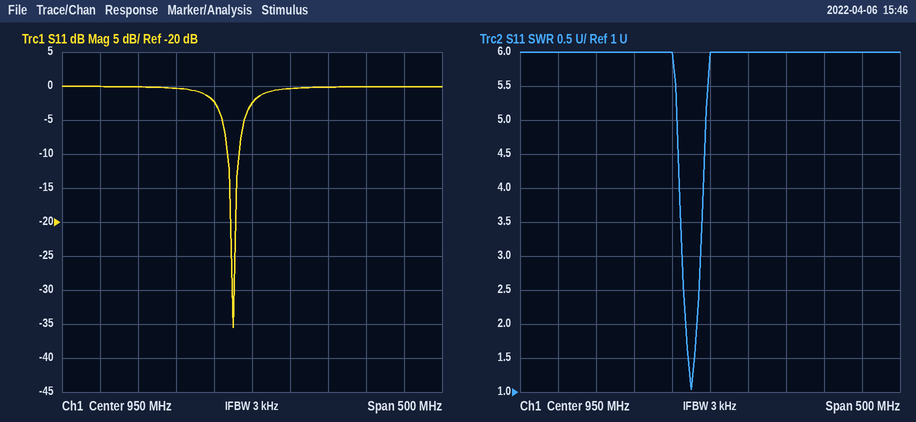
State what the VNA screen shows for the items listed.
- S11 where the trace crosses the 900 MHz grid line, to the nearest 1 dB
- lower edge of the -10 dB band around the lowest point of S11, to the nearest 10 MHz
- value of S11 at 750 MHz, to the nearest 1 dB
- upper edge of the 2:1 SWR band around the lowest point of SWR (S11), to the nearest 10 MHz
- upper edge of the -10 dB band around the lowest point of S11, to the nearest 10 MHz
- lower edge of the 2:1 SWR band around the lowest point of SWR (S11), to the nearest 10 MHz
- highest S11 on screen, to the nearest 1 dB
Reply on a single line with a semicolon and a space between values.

-2 dB; 920 MHz; 0 dB; 930 MHz; 930 MHz; 920 MHz; 0 dB
